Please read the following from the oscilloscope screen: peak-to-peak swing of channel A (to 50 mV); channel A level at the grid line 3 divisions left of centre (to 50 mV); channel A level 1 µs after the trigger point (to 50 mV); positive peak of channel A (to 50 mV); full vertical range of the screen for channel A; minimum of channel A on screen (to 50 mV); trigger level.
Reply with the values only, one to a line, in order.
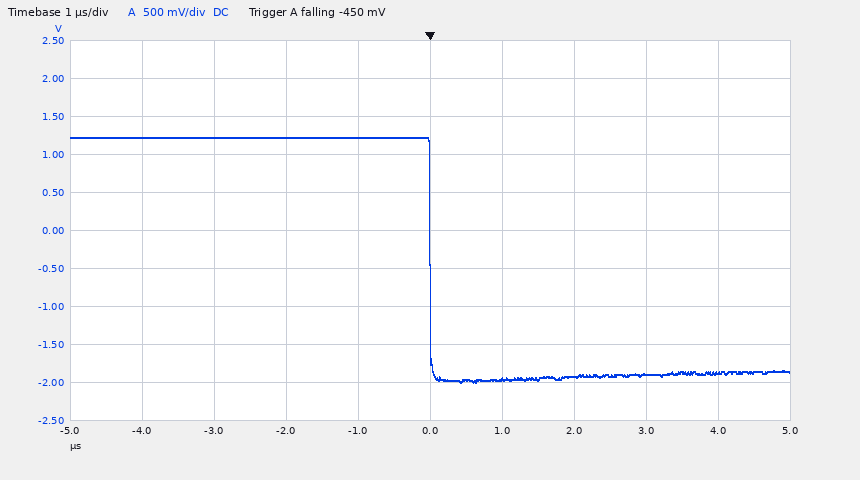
3.20 V
1.20 V
-1.95 V
1.20 V
5 V
-2.00 V
-450 mV
